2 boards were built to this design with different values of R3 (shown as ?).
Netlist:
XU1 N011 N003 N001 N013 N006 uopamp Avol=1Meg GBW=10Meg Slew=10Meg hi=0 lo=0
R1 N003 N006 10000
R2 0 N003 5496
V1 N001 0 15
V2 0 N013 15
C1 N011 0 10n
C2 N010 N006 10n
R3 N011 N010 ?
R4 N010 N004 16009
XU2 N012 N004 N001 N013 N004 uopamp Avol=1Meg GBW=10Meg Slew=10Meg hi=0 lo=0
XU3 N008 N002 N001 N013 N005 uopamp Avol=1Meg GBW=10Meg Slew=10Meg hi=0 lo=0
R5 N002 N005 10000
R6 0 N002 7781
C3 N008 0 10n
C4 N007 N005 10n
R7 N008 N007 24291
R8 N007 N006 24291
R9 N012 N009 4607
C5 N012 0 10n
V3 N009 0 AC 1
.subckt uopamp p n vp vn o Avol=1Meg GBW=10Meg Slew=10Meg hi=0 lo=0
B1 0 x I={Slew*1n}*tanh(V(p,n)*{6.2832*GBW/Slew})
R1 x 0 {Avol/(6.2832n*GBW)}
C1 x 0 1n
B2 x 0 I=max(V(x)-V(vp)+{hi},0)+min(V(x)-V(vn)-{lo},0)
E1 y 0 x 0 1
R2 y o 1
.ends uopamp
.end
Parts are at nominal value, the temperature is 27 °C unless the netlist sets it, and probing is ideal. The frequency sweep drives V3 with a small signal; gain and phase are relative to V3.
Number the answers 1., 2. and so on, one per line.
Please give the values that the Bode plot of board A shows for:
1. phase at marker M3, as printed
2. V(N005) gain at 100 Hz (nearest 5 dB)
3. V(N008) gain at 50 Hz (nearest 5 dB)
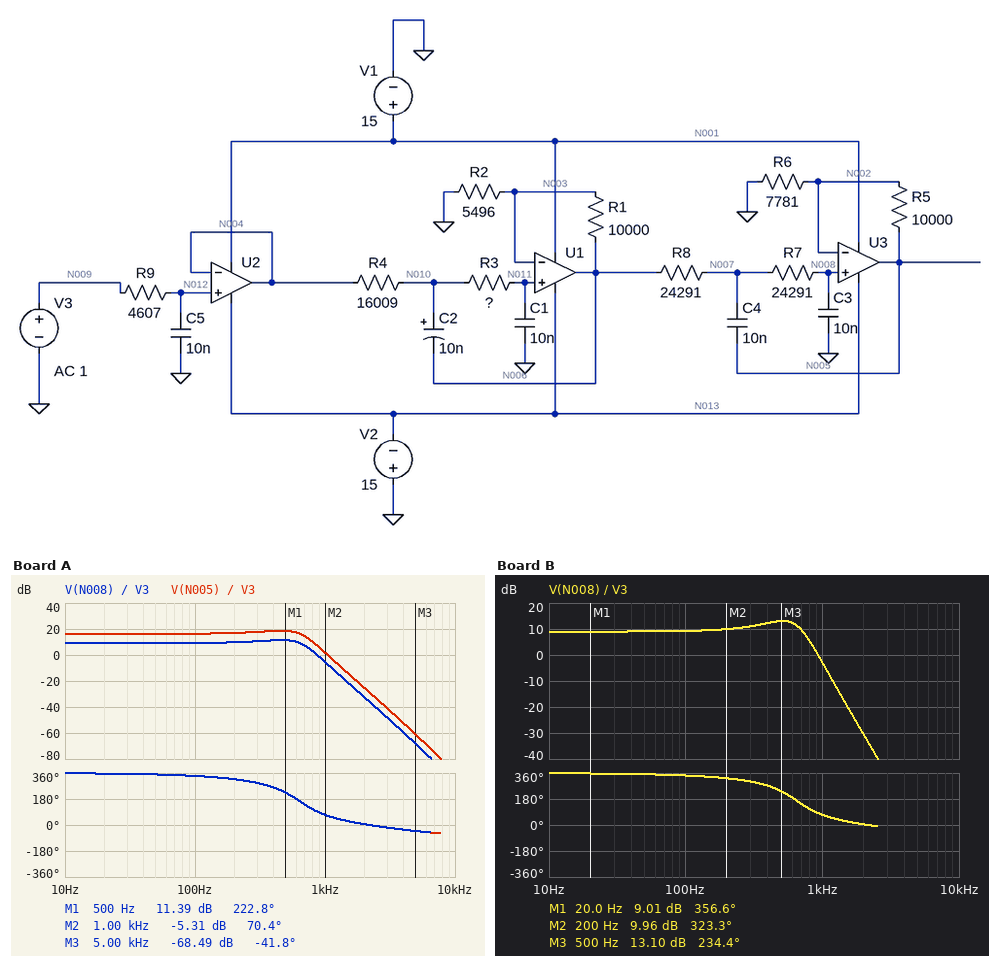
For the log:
1. -41.8 deg
2. 15 dB
3. 10 dB
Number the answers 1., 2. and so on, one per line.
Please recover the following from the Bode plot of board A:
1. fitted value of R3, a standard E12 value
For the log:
1. 47 kΩ
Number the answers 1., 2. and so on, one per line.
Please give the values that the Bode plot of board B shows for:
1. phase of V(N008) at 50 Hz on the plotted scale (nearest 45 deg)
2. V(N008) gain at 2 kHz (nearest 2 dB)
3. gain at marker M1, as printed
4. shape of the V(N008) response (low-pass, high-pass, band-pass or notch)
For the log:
1. 360 deg
2. -30 dB
3. 9.01 dB
4. low-pass
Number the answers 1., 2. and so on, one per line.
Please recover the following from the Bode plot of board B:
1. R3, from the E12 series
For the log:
1. 39 kΩ
